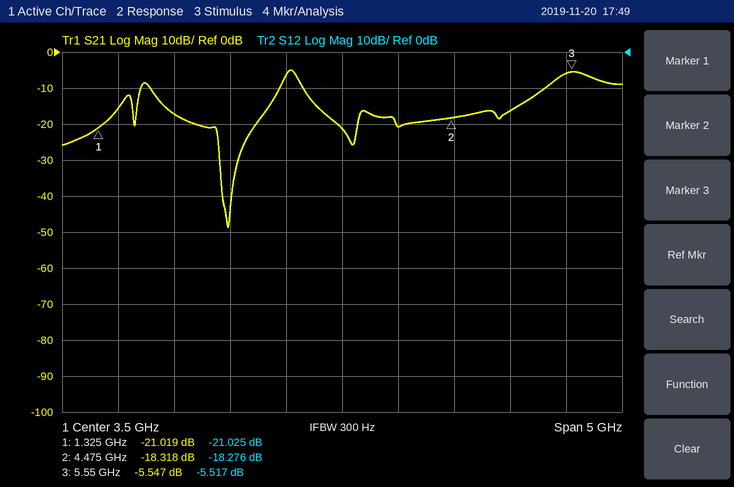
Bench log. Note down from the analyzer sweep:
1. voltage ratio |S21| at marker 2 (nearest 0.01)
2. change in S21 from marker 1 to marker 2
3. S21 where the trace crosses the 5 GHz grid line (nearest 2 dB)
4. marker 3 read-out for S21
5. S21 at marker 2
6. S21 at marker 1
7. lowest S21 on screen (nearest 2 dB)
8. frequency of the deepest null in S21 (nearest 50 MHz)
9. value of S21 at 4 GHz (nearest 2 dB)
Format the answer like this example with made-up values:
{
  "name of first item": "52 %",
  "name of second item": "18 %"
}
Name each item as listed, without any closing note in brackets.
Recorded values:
{
  "voltage ratio |S21| at marker 2": "0.12",
  "change in S21 from marker 1 to marker 2": "2.701 dB",
  "S21 where the trace crosses the 5 GHz grid line": "-16 dB",
  "marker 3 read-out for S21": "-5.547 dB",
  "S21 at marker 2": "-18.318 dB",
  "S21 at marker 1": "-21.019 dB",
  "lowest S21 on screen": "-48 dB",
  "frequency of the deepest null in S21": "2.50 GHz",
  "value of S21 at 4 GHz": "-20 dB"
}
